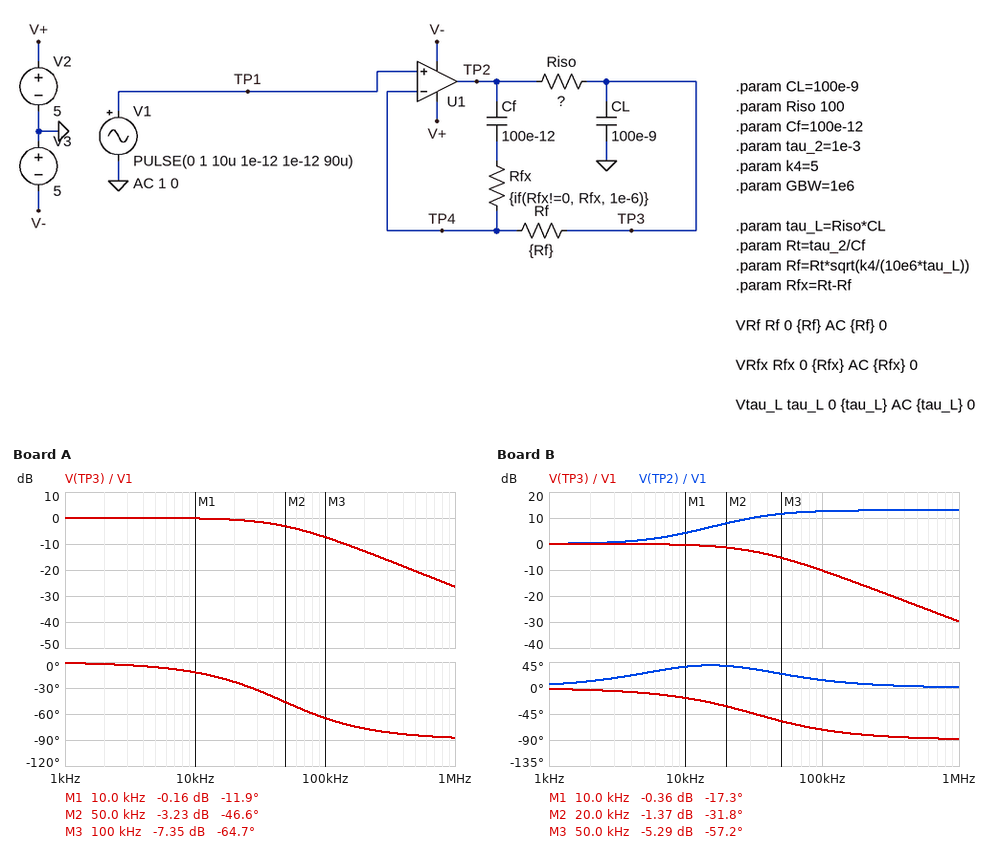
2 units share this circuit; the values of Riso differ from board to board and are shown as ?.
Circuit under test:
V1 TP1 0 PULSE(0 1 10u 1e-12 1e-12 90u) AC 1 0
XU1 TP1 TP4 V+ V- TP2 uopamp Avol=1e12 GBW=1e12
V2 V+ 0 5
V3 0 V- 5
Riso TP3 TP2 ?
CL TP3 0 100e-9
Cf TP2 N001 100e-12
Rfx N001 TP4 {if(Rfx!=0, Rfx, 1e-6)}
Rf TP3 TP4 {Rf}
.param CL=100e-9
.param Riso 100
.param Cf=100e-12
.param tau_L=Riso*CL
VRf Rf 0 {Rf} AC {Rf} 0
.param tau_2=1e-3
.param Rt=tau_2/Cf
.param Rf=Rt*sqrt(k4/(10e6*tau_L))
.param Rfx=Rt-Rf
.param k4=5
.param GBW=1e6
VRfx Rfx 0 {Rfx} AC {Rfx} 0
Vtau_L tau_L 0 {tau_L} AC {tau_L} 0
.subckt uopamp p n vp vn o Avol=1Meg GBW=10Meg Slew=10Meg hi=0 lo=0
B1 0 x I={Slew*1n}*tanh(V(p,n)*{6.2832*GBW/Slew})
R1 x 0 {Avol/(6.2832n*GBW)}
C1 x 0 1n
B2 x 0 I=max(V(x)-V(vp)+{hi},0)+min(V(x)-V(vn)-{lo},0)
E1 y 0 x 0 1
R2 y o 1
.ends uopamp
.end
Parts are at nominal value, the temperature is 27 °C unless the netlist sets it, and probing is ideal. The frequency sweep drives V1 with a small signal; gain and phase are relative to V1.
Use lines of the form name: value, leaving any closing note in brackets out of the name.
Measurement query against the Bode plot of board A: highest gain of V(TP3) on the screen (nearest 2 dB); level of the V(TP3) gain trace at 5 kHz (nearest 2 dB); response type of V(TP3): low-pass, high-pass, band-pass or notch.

highest gain of V(TP3) on the screen: 0 dB
level of the V(TP3) gain trace at 5 kHz: 0 dB
response type of V(TP3): low-pass, high-pass, band-pass or notch: low-pass
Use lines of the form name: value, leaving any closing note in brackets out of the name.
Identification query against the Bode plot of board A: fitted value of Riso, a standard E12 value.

fitted value of Riso, a standard E12 value: 150 Ω
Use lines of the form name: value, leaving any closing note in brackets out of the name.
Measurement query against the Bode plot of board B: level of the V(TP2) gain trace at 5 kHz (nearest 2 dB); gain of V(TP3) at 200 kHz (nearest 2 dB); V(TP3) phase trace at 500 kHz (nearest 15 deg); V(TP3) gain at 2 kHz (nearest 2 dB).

level of the V(TP2) gain trace at 5 kHz: 2 dB
gain of V(TP3) at 200 kHz: -16 dB
V(TP3) phase trace at 500 kHz: -90 deg
V(TP3) gain at 2 kHz: 0 dB
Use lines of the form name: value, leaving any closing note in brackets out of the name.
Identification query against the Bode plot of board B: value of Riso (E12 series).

value of Riso: 220 Ω
